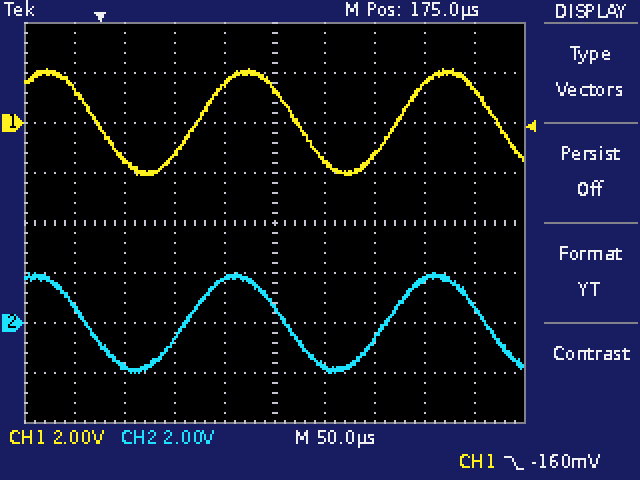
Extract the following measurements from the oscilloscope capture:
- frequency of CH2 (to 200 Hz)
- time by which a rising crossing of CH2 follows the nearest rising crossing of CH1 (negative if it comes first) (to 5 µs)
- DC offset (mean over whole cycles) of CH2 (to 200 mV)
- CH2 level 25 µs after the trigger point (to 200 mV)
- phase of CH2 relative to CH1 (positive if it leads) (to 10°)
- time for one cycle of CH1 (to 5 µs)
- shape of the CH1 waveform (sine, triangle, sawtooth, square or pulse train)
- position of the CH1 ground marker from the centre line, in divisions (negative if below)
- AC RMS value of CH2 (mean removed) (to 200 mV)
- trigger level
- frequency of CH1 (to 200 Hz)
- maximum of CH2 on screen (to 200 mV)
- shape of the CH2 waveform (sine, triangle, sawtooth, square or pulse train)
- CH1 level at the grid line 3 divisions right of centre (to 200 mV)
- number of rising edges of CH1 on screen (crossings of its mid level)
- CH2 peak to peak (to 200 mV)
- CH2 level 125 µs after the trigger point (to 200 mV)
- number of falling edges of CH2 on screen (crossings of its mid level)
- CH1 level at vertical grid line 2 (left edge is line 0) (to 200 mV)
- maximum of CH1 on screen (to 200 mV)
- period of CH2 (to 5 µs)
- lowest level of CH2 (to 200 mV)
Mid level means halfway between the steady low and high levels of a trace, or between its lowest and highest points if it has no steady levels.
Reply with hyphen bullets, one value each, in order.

- 5.0 kHz
- -10 µs
- 0.0 V
- -1.8 V
- +20°
- 200 µs
- sine
- +2.0 div
- 1.4 V
- -160 mV
- 5.0 kHz
- 2.0 V
- sine
- 1.6 V
- 2
- 4.0 V
- 1.8 V
- 3
- -1.4 V
- 2.2 V
- 200 µs
- -2.0 V
